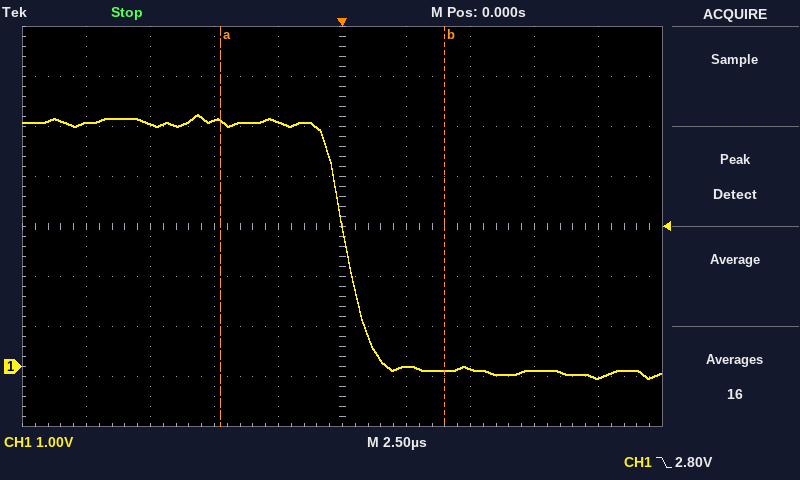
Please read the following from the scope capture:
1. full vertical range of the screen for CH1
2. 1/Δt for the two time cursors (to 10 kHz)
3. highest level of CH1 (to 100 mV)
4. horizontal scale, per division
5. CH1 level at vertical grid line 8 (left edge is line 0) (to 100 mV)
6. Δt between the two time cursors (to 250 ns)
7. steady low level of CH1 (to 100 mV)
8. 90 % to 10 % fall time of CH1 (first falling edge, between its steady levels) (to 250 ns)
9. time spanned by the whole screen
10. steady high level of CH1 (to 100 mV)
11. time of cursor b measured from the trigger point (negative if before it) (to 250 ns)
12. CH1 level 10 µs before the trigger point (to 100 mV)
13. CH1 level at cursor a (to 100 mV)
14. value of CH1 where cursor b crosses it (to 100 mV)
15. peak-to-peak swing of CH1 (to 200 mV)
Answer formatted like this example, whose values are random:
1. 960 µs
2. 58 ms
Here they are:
1. 8 V
2. 110 kHz
3. 5.0 V
4. 2.5 µs
5. -100 mV
6. 8.75 µs
7. -100 mV
8. 1.75 µs
9. 25 µs
10. 4.9 V
11. +4.00 µs
12. 4.9 V
13. 4.9 V
14. -100 mV
15. 5.2 V
